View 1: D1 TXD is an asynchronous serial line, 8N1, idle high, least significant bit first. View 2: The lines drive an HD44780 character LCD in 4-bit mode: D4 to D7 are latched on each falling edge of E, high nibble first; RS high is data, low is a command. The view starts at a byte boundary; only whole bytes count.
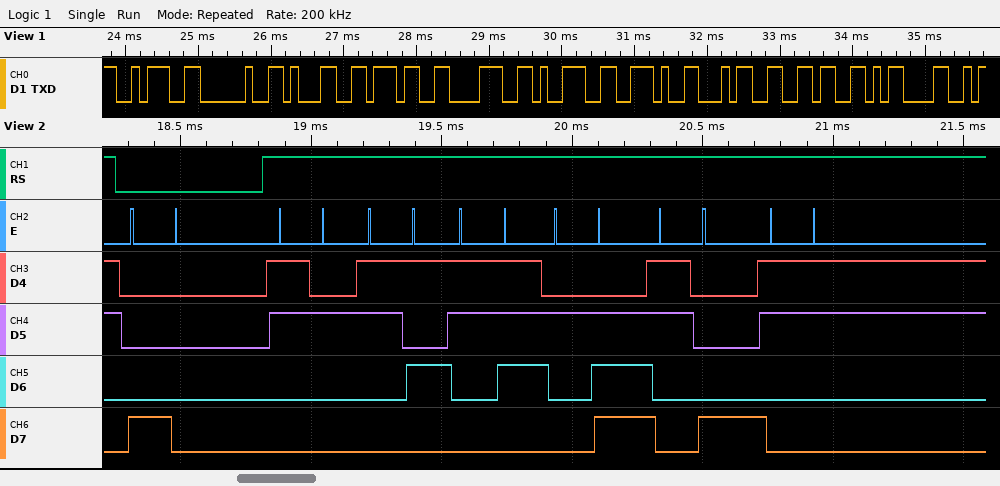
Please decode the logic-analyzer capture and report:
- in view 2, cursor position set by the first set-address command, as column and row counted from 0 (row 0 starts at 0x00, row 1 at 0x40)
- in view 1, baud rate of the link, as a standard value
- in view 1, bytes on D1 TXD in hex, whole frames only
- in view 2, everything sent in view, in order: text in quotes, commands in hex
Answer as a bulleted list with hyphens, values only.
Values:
- column 0, row 0
- 9600 baud
- 3A 20 31 37 38 39 2E 34 36 0D
- 0x80 "257.83"
